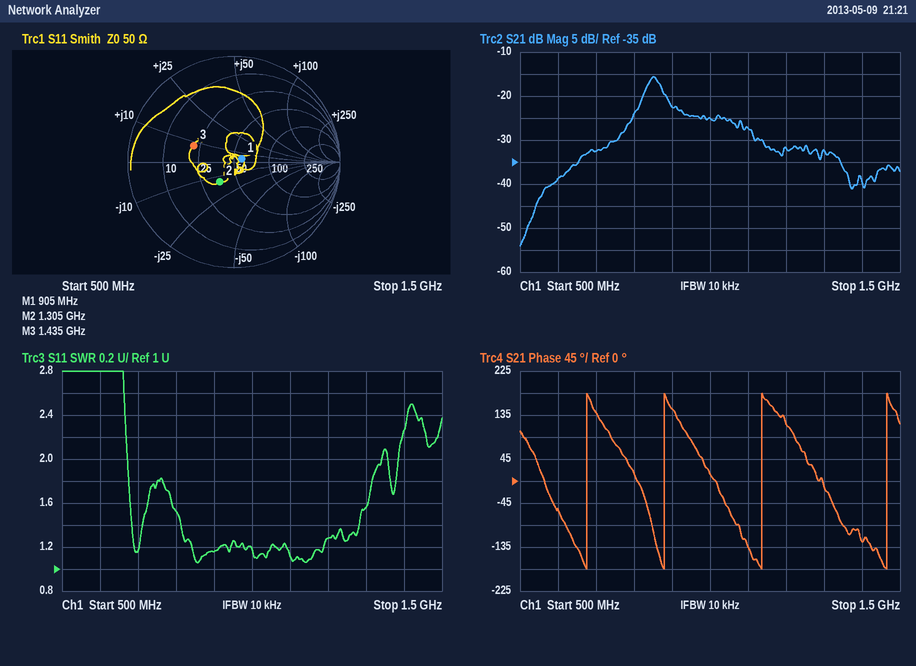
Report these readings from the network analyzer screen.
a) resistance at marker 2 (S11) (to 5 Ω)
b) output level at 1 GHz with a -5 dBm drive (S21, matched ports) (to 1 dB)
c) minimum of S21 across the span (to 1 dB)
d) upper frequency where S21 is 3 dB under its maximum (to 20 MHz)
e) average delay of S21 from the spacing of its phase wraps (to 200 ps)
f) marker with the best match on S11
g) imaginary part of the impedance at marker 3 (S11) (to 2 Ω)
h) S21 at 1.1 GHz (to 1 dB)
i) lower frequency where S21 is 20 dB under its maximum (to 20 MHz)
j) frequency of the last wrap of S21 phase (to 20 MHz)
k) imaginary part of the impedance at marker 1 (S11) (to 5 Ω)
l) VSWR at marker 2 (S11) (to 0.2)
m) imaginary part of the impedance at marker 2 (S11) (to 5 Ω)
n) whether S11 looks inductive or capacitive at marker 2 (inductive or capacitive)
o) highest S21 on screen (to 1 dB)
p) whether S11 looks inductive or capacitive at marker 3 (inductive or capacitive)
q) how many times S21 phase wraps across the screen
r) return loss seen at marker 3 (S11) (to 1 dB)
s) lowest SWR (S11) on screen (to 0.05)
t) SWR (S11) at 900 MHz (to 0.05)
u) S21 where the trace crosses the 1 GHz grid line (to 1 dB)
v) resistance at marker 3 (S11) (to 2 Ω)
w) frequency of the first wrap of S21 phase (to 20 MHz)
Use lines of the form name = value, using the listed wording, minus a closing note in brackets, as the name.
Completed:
resistance at marker 2 (S11) = 35 Ω
output level at 1 GHz with a -5 dBm drive (S21, matched ports) = -30 dBm
minimum of S21 across the span = -54 dB
upper frequency where S21 is 3 dB under its maximum = 880 MHz
average delay of S21 from the spacing of its phase wraps = 3.8 ns
marker with the best match on S11 = marker 1
imaginary part of the impedance at marker 3 (S11) = +8 Ω
S21 at 1.1 GHz = -27 dB
lower frequency where S21 is 20 dB under its maximum = 640 MHz
frequency of the last wrap of S21 phase = 1.46 GHz
imaginary part of the impedance at marker 1 (S11) = +5 Ω
VSWR at marker 2 (S11) = 1.6
imaginary part of the impedance at marker 2 (S11) = -15 Ω
whether S11 looks inductive or capacitive at marker 2 = capacitive
highest S21 on screen = -16 dB
whether S11 looks inductive or capacitive at marker 3 = inductive
how many times S21 phase wraps across the screen = 4
return loss seen at marker 3 (S11) = 8 dB
lowest SWR (S11) on screen = 1.05
SWR (S11) at 900 MHz = 1.15
S21 where the trace crosses the 1 GHz grid line = -25 dB
resistance at marker 3 (S11) = 22 Ω
frequency of the first wrap of S21 phase = 680 MHz
